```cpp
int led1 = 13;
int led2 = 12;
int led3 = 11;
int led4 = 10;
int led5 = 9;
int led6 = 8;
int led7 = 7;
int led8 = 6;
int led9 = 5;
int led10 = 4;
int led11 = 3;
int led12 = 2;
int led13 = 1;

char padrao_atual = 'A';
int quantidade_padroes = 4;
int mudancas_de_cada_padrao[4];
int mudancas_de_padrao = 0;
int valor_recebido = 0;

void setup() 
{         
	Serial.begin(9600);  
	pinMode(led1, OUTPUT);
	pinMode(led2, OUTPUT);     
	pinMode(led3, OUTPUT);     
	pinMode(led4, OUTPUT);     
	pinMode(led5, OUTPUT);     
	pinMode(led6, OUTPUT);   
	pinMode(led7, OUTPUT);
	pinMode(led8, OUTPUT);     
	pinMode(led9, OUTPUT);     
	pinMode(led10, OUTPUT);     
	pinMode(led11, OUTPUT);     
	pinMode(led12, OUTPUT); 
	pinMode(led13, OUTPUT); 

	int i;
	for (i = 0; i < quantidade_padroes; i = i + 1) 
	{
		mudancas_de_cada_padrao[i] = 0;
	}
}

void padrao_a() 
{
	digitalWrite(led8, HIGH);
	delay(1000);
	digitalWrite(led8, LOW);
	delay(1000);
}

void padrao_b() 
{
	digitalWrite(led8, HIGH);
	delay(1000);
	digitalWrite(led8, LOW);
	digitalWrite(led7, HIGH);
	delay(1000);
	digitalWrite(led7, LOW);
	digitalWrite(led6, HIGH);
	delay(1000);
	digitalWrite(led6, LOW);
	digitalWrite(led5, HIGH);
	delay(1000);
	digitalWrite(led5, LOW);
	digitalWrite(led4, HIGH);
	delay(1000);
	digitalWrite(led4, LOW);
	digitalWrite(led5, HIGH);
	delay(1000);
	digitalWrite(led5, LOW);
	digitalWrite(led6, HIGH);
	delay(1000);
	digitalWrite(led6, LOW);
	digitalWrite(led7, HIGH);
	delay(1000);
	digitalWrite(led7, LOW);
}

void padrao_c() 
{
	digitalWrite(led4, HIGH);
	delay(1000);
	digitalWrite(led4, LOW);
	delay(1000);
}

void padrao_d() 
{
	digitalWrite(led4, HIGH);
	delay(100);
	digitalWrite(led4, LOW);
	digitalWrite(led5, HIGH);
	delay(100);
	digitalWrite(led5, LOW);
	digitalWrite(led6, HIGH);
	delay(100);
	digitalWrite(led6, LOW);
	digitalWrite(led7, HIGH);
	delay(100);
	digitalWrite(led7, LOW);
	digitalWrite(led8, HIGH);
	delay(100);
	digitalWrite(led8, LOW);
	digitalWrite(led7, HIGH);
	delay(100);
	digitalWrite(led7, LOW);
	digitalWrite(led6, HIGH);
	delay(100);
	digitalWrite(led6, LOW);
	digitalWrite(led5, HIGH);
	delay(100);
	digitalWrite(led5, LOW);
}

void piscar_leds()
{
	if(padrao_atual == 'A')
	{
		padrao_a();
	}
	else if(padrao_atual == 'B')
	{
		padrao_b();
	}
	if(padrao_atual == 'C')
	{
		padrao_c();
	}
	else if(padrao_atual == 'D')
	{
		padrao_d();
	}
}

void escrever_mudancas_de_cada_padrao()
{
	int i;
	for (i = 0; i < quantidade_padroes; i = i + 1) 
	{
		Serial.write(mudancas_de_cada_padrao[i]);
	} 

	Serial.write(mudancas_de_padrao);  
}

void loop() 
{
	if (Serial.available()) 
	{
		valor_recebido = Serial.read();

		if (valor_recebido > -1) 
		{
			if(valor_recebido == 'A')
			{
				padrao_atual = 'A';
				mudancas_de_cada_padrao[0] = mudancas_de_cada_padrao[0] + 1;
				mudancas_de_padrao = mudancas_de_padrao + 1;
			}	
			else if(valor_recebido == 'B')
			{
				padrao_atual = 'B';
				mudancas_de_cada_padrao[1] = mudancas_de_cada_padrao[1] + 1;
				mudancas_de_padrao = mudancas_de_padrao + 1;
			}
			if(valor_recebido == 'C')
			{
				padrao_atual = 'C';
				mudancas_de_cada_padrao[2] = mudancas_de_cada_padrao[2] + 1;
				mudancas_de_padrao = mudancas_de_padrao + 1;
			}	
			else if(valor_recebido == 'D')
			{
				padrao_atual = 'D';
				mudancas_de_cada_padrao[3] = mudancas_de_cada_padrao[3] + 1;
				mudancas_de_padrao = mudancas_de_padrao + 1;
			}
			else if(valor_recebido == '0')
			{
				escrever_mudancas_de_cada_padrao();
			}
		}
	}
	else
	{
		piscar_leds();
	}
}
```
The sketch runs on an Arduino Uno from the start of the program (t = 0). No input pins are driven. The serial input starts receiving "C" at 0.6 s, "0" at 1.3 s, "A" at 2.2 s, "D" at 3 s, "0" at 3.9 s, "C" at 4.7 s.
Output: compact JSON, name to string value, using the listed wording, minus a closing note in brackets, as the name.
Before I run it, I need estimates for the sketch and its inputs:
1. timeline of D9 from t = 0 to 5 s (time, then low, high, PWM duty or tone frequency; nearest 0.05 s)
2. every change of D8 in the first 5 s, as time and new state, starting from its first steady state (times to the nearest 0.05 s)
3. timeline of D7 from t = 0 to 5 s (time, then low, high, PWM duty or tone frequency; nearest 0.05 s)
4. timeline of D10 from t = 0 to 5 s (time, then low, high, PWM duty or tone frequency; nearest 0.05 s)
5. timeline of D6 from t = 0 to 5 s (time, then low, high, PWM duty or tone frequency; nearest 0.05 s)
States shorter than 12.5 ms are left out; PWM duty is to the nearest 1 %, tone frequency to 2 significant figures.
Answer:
{"timeline of D9 from t = 0 to 5 s": "0 s low; 4.1 s high; 4.2 s low; 4.7 s high; 4.8 s low", "every change of D8 in the first 5 s, as time and new state, starting from its first steady state": "0 s low; 4.2 s high; 4.3 s low; 4.6 s high; 4.7 s low", "timeline of D7 from t = 0 to 5 s": "0 s low; 4.3 s high; 4.4 s low; 4.5 s high; 4.6 s low", "timeline of D10 from t = 0 to 5 s": "0 s low; 2 s high; 3 s low; 4 s high; 4.1 s low; 4.8 s high", "timeline of D6 from t = 0 to 5 s": "0 s high; 1 s low; 4.4 s high; 4.5 s low"}
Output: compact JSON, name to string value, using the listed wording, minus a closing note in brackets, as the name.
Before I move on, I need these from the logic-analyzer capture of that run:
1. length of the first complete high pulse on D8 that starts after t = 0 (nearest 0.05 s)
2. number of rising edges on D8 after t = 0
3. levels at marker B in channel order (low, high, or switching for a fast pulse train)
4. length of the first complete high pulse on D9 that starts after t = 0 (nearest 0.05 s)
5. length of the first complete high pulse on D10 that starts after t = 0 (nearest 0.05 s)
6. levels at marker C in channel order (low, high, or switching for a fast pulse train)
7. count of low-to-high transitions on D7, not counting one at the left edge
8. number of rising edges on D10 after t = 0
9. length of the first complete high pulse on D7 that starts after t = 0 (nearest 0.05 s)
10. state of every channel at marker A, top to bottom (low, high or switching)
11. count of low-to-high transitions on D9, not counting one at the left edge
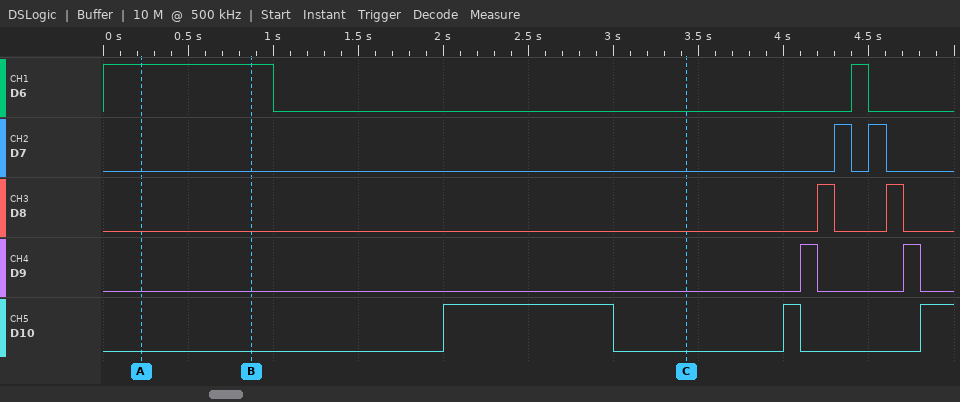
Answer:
{"length of the first complete high pulse on D8 that starts after t = 0": "0.10 s", "number of rising edges on D8 after t = 0": "2", "levels at marker B in channel order": "D6 high, D7 low, D8 low, D9 low, D10 low", "length of the first complete high pulse on D9 that starts after t = 0": "0.10 s", "length of the first complete high pulse on D10 that starts after t = 0": "1.00 s", "levels at marker C in channel order": "D6 low, D7 low, D8 low, D9 low, D10 low", "count of low-to-high transitions on D7, not counting one at the left edge": "2", "number of rising edges on D10 after t = 0": "3", "length of the first complete high pulse on D7 that starts after t = 0": "0.10 s", "state of every channel at marker A, top to bottom": "D6 high, D7 low, D8 low, D9 low, D10 low", "count of low-to-high transitions on D9, not counting one at the left edge": "2"}
